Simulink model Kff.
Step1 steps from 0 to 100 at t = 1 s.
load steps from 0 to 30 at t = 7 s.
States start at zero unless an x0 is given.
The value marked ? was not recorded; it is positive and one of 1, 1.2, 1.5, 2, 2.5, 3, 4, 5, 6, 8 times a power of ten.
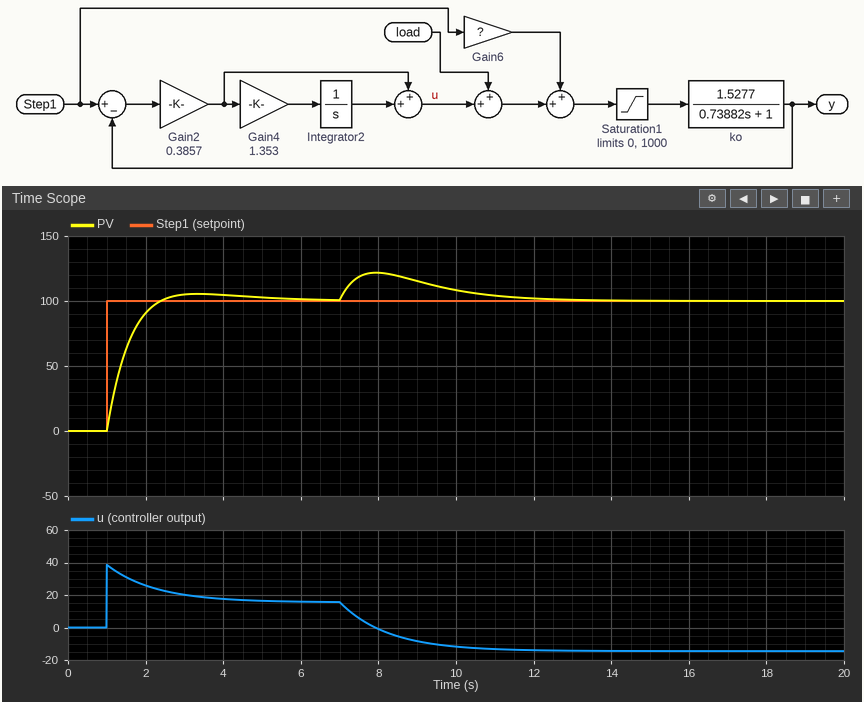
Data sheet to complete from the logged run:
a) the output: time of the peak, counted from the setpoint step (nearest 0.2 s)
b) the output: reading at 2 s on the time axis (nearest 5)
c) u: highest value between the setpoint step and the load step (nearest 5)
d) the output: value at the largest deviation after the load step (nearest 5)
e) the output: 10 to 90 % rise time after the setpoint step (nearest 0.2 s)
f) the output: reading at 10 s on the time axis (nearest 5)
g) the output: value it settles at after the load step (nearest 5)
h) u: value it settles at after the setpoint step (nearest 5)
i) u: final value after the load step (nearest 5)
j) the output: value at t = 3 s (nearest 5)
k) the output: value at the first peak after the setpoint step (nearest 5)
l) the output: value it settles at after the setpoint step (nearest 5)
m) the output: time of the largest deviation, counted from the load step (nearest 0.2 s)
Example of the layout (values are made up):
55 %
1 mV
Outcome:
2.4 s
90
40
120
1.0 s
110
100
15
-15
105
105
100
1.0 s
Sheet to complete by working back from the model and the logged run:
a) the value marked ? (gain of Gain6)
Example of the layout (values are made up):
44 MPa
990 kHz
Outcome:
0.5
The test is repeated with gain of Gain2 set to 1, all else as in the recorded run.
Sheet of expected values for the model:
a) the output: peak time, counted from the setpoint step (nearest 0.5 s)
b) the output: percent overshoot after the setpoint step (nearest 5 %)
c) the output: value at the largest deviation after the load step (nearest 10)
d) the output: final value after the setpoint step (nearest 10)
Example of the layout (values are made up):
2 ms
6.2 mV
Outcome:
1.5 s
10 %
110
100
